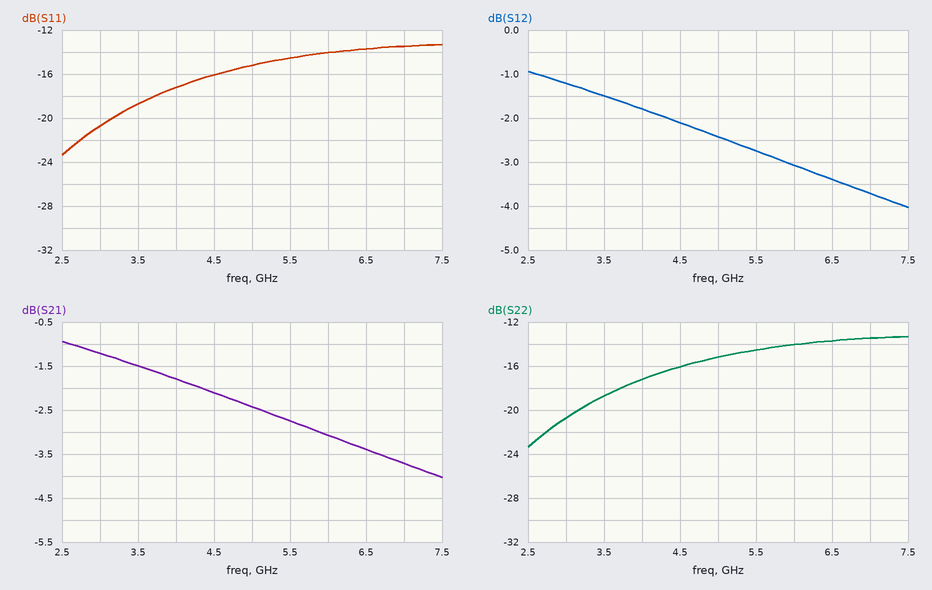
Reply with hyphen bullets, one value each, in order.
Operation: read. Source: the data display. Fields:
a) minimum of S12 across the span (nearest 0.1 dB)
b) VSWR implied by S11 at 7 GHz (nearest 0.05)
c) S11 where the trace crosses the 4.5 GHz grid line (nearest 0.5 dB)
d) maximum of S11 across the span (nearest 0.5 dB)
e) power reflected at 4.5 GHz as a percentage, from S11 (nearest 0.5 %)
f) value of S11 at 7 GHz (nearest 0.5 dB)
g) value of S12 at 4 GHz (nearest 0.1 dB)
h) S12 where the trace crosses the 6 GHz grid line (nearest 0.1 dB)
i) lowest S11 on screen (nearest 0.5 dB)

- -4.0 dB
- 1.55
- -16.0 dB
- -13.5 dB
- 2.5 %
- -13.5 dB
- -1.8 dB
- -3.1 dB
- -23.5 dB
